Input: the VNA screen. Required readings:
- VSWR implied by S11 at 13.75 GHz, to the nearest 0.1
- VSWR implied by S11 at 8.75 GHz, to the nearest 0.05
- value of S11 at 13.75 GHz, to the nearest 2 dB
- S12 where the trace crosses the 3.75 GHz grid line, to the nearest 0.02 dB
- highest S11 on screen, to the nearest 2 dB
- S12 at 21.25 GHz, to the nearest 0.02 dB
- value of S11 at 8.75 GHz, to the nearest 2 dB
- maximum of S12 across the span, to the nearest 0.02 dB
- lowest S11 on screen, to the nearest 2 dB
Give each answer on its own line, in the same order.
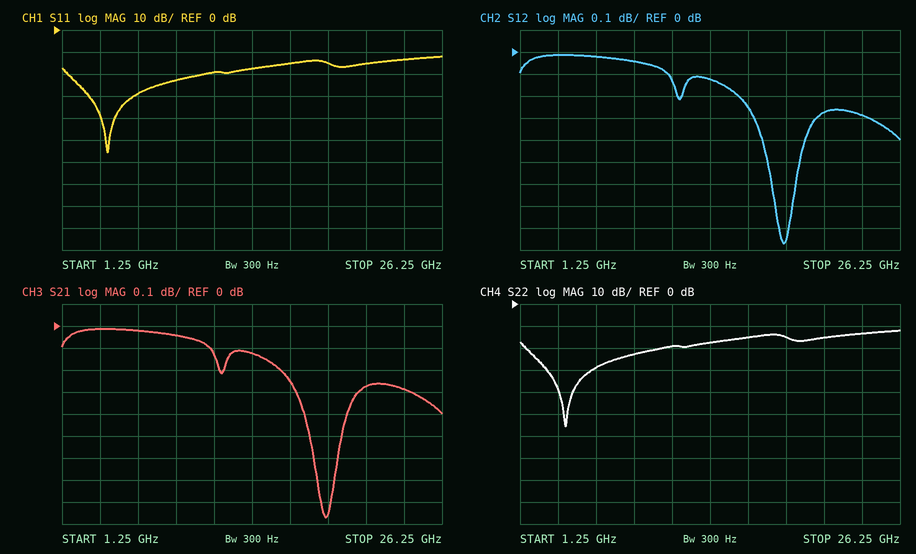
1.3
1.15
-18 dB
-0.02 dB
-12 dB
-0.28 dB
-22 dB
-0.02 dB
-56 dB
